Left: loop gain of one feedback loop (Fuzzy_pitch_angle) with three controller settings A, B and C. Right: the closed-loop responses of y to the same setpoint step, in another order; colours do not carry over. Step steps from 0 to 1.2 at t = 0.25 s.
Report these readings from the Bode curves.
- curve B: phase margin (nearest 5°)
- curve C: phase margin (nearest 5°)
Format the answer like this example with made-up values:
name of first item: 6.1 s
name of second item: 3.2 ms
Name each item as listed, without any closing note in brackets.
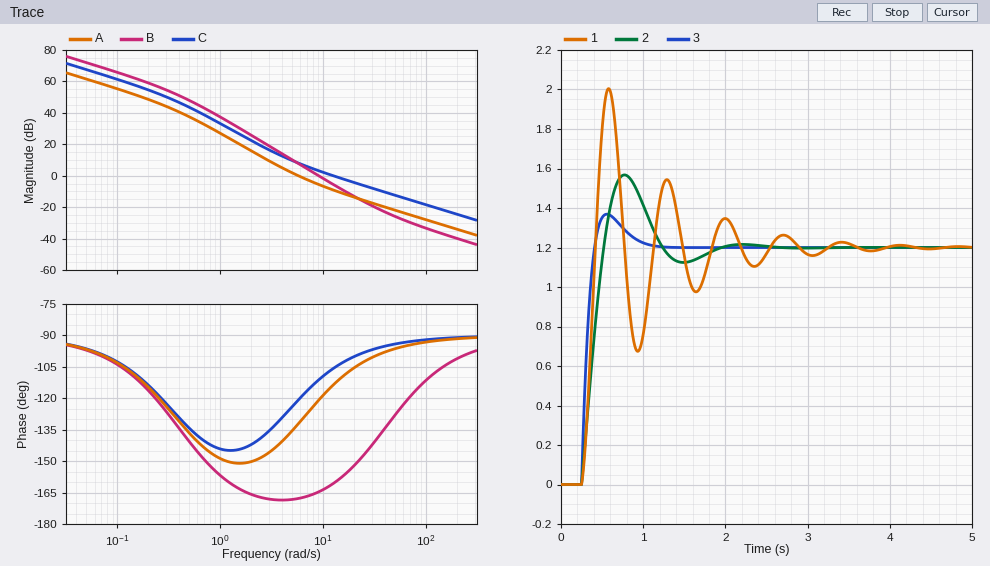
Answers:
curve B: phase margin: 15°
curve C: phase margin: 75°
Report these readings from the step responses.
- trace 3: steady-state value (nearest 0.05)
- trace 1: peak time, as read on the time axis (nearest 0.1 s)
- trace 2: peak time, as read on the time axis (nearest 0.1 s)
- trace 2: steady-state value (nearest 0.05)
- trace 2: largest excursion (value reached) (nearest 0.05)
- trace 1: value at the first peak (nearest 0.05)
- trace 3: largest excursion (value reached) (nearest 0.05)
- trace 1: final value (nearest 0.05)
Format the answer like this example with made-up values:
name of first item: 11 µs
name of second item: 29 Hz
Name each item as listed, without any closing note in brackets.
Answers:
trace 3: steady-state value: 1.20
trace 1: peak time, as read on the time axis: 0.6 s
trace 2: peak time, as read on the time axis: 0.8 s
trace 2: steady-state value: 1.20
trace 2: largest excursion (value reached): 1.55
trace 1: value at the first peak: 2.00
trace 3: largest excursion (value reached): 1.35
trace 1: final value: 1.20
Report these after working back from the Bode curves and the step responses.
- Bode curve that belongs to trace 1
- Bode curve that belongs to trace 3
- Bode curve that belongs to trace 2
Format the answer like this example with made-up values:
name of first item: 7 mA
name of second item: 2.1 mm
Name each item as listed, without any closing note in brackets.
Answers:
Bode curve that belongs to trace 1: B
Bode curve that belongs to trace 3: C
Bode curve that belongs to trace 2: A
